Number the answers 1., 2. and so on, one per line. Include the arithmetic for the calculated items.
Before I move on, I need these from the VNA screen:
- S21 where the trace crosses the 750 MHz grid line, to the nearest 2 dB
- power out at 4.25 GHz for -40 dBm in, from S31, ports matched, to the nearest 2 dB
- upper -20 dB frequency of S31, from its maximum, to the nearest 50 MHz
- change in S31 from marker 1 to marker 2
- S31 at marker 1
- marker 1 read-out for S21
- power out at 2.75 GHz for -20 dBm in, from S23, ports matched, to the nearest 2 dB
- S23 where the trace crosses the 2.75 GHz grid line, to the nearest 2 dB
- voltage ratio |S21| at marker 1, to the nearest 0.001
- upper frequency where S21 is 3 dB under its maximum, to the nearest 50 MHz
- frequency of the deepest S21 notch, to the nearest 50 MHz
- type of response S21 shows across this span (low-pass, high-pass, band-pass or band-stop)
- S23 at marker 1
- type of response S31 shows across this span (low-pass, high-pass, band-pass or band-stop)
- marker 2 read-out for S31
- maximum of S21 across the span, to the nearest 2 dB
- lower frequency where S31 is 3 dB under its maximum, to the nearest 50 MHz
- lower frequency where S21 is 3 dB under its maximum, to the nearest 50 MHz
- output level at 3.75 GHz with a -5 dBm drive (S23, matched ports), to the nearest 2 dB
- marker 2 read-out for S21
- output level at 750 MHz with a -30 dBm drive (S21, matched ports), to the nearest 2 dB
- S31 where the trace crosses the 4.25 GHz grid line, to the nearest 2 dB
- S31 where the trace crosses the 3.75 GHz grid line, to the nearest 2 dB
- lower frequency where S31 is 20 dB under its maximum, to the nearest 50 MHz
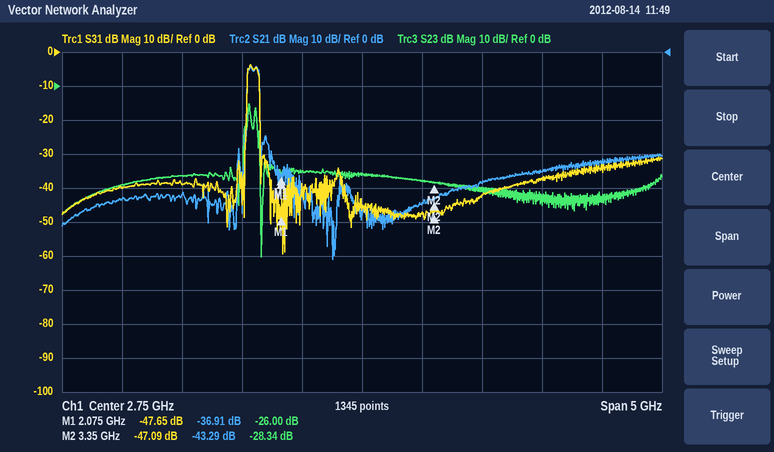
1. -44 dB
2. -40 dBm + (-38 dB) = -78 dBm
3. 1.90 GHz
4. -47.09 − (-47.65) = 0.56 dB
5. -47.65 dB
6. -36.91 dB
7. -20 dBm + (-26 dB) = -46 dBm
8. -26 dB
9. 10^(-36.91/20) ≈ 0.014
10. 1.90 GHz
11. 2.50 GHz
12. band-pass
13. -26.00 dB
14. band-pass
15. -47.09 dB
16. -4 dB
17. 1.80 GHz
18. 1.80 GHz
19. -5 dBm + (-30 dB) = -36 dBm
20. -43.29 dB
21. -30 dBm + (-44 dB) = -74 dBm
22. -38 dB
23. -42 dB
24. 1.80 GHz
